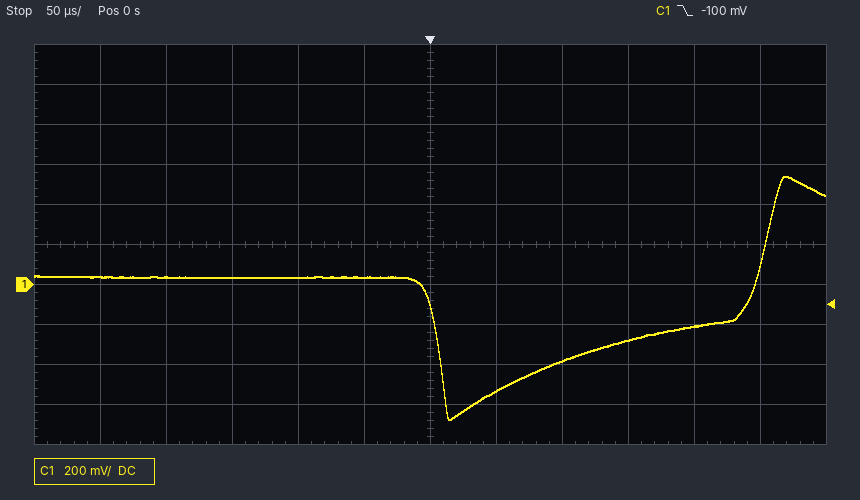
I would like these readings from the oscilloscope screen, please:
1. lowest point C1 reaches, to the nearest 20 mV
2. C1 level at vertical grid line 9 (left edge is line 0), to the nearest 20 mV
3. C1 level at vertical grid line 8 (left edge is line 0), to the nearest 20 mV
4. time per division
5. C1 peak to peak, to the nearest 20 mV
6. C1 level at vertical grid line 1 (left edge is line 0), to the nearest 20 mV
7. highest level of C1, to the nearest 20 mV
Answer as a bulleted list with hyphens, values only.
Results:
- -680 mV
- -280 mV
- -380 mV
- 50 µs
- 1.22 V
- 40 mV
- 540 mV
